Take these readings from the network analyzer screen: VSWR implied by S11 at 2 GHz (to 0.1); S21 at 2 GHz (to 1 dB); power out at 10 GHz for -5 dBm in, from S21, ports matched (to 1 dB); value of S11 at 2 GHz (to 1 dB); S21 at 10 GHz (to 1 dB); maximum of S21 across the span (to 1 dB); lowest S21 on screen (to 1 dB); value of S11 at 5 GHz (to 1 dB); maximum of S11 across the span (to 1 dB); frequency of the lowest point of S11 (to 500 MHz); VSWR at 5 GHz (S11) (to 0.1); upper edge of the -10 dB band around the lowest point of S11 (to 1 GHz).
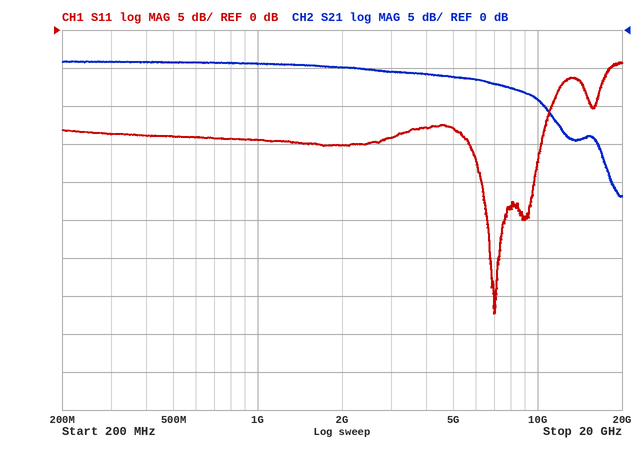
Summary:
1.4
-5 dB
-14 dBm
-15 dB
-9 dB
-4 dB
-22 dB
-13 dB
-4 dB
7.0 GHz
1.6
11 GHz
